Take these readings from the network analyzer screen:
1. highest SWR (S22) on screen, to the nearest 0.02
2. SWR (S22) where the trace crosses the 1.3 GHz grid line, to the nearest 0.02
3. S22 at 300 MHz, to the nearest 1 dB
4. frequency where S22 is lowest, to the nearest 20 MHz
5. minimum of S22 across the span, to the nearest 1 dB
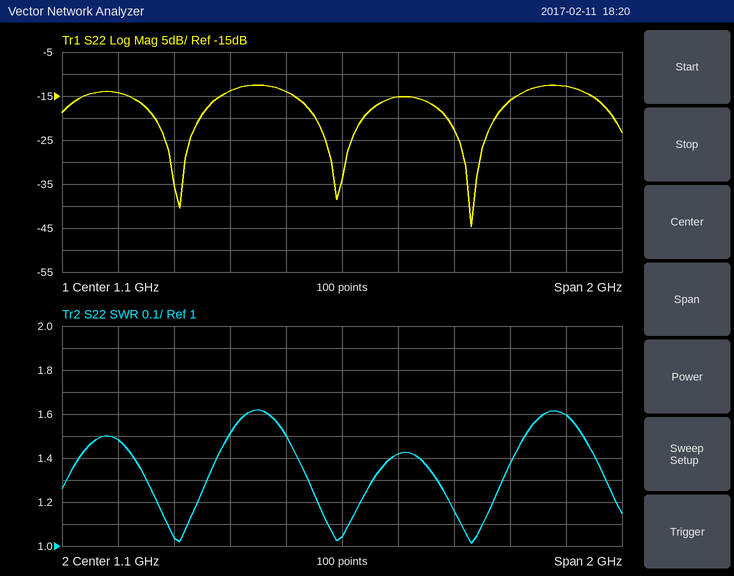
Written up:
1.62
1.42
-14 dB
1.56 GHz
-45 dB
